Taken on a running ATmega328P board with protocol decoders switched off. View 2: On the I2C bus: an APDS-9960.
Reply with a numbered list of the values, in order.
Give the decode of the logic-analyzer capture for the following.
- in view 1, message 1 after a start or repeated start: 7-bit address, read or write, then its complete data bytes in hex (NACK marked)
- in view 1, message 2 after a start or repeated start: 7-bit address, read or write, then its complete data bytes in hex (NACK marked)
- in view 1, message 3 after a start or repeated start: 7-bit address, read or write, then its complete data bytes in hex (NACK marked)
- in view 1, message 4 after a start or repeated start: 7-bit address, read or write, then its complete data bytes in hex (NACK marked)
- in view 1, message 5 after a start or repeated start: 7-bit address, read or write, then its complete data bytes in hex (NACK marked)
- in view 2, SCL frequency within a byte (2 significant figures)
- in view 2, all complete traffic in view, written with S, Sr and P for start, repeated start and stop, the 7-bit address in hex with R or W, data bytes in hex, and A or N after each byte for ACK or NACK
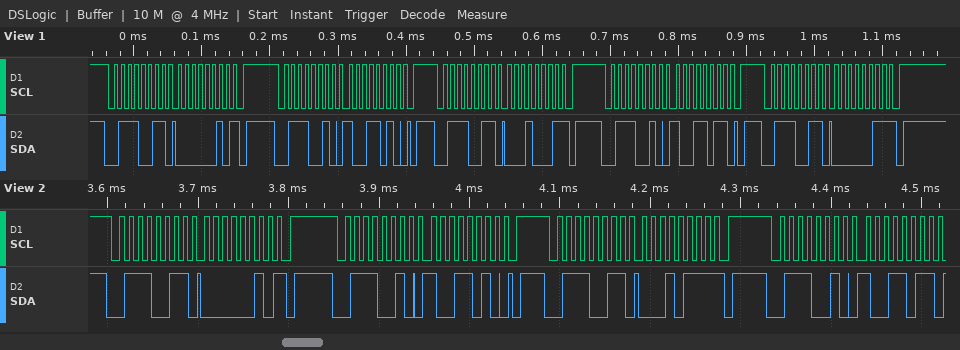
1. 0x39 read: 02 NACK
2. 0x39 write: 9A
3. 0x39 read: 11 NACK
4. 0x39 write: 9B
5. 0x39 read: 03 NACK
6. 100 kHz
7. S 39R A 02 N P S 39W A 9A A P S 39R A 17 N P S 39W A 9B A
